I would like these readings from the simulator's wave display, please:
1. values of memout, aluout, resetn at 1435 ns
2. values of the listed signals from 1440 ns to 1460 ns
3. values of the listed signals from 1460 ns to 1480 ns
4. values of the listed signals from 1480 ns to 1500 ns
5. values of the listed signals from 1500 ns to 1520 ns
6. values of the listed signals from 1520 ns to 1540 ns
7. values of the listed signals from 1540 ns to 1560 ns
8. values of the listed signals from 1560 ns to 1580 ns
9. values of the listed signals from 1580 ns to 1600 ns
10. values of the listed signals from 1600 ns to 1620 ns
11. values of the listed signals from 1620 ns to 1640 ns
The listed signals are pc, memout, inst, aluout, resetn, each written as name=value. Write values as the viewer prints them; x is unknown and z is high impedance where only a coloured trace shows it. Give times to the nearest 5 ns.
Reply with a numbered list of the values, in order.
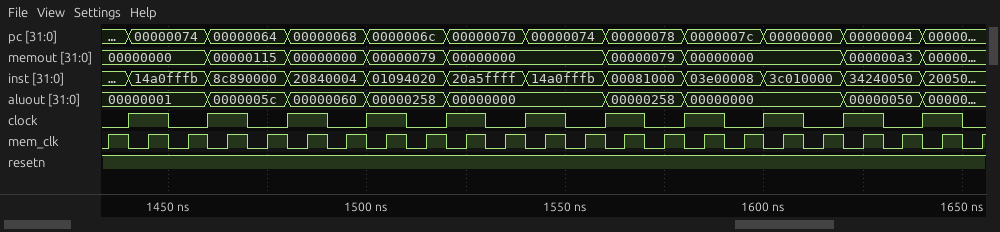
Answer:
1. memout=00000000, aluout=00000001, resetn=1
2. pc=00000074, memout=00000000, inst=14a0fffb, aluout=00000001, resetn=1
3. pc=00000064, memout=00000115, inst=8c890000, aluout=0000005c, resetn=1
4. pc=00000068, memout=00000000, inst=20840004, aluout=00000060, resetn=1
5. pc=0000006c, memout=00000079, inst=01094020, aluout=00000258, resetn=1
6. pc=00000070, memout=00000000, inst=20a5ffff, aluout=00000000, resetn=1
7. pc=00000074, memout=00000000, inst=14a0fffb, aluout=00000000, resetn=1
8. pc=00000078, memout=00000079, inst=00081000, aluout=00000258, resetn=1
9. pc=0000007c, memout=00000000, inst=03e00008, aluout=00000000, resetn=1
10. pc=00000000, memout=00000000, inst=3c010000, aluout=00000000, resetn=1
11. pc=00000004, memout=000000a3, inst=34240050, aluout=00000050, resetn=1
